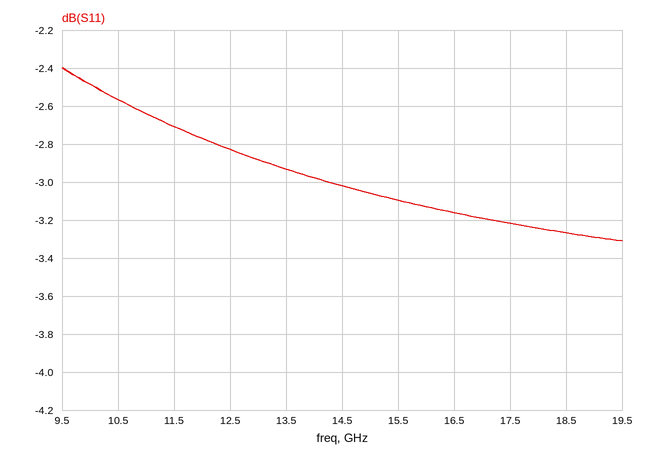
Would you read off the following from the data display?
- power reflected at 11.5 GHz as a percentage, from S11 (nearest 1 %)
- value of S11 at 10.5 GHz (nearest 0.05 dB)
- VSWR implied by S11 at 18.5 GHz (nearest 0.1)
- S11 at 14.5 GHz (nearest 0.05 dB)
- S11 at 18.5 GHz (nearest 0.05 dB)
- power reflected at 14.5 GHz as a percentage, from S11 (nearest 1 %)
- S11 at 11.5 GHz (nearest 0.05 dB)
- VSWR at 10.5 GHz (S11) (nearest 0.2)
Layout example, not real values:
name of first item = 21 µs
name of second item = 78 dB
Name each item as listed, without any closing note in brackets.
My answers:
power reflected at 11.5 GHz as a percentage, from S11 = 54 %
value of S11 at 10.5 GHz = -2.55 dB
VSWR implied by S11 at 18.5 GHz = 5.4
S11 at 14.5 GHz = -3.00 dB
S11 at 18.5 GHz = -3.25 dB
power reflected at 14.5 GHz as a percentage, from S11 = 50 %
S11 at 11.5 GHz = -2.70 dB
VSWR at 10.5 GHz (S11) = 6.8
